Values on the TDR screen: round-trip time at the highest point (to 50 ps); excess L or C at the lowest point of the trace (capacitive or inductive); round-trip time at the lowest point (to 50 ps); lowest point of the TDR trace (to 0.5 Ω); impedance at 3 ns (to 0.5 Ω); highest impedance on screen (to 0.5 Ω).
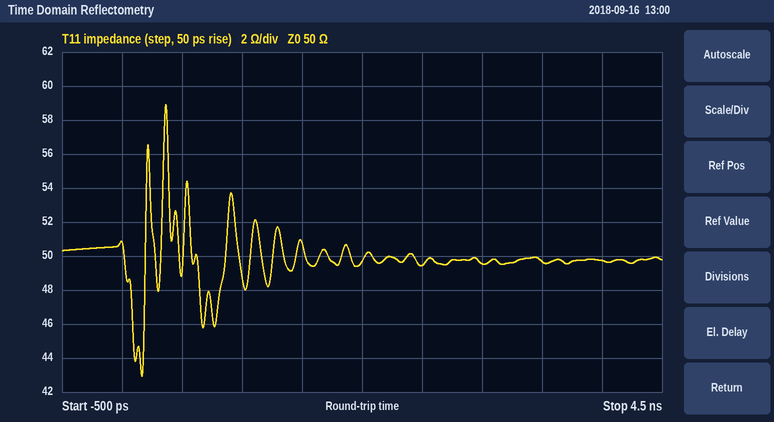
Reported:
350 ps
capacitive
150 ps
43.0 Ω
49.5 Ω
59.0 Ω
